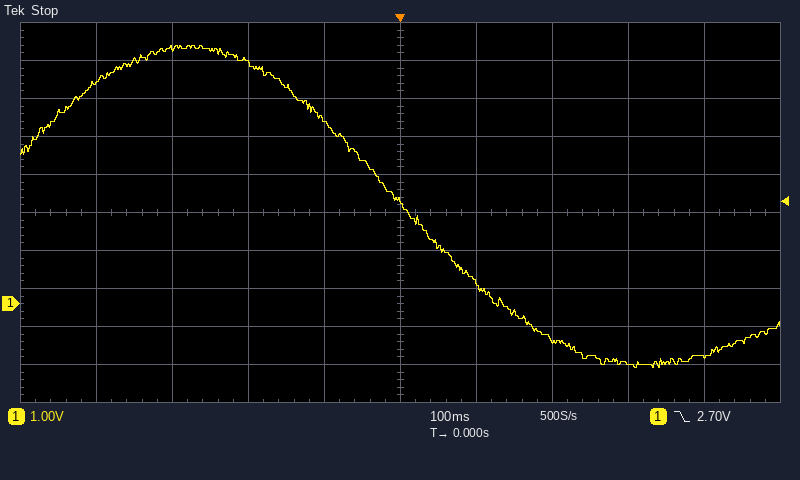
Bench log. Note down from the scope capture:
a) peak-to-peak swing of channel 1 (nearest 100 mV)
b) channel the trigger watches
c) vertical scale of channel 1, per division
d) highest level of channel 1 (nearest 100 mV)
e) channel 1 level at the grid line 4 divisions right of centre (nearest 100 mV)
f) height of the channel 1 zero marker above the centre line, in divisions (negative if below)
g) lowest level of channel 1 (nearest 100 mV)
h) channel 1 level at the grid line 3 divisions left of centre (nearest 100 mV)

8.5 V
channel 1
1 V
6.8 V
-1.4 V
-2.4 div
-1.7 V
6.7 V
